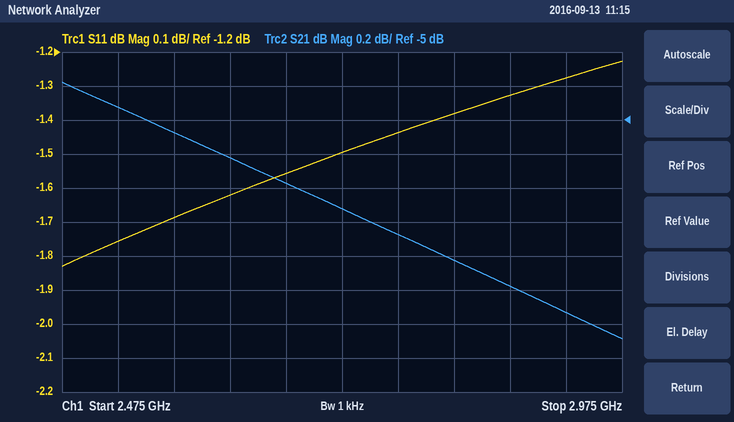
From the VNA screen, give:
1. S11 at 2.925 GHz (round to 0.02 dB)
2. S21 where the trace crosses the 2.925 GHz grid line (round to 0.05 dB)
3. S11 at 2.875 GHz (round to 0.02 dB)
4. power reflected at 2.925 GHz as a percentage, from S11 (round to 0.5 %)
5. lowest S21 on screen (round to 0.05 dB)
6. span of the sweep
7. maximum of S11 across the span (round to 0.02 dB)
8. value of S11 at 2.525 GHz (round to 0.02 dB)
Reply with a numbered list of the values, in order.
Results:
1. -1.28 dB
2. -6.15 dB
3. -1.32 dB
4. 74.5 %
5. -6.30 dB
6. 500 MHz
7. -1.22 dB
8. -1.76 dB
